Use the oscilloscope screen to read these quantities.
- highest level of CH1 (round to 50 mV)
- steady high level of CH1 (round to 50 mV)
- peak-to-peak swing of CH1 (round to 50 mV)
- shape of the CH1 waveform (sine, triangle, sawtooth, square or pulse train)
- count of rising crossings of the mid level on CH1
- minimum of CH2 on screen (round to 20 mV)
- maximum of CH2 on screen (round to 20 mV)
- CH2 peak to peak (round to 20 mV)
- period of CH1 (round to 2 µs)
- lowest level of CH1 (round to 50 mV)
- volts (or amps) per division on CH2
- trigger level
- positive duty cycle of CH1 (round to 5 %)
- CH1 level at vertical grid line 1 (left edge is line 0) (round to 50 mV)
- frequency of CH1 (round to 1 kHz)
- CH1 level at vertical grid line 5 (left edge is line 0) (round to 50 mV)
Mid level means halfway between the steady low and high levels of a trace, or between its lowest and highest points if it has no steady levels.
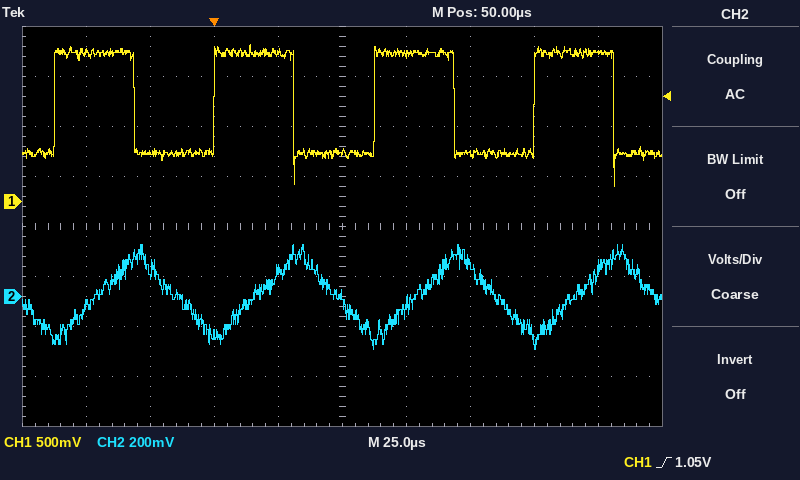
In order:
1.55 V
1.50 V
1.40 V
square
4
-220 mV
200 mV
420 mV
62 µs
150 mV
200 mV
1.05 V
50 %
1.50 V
16 kHz
500 mV
